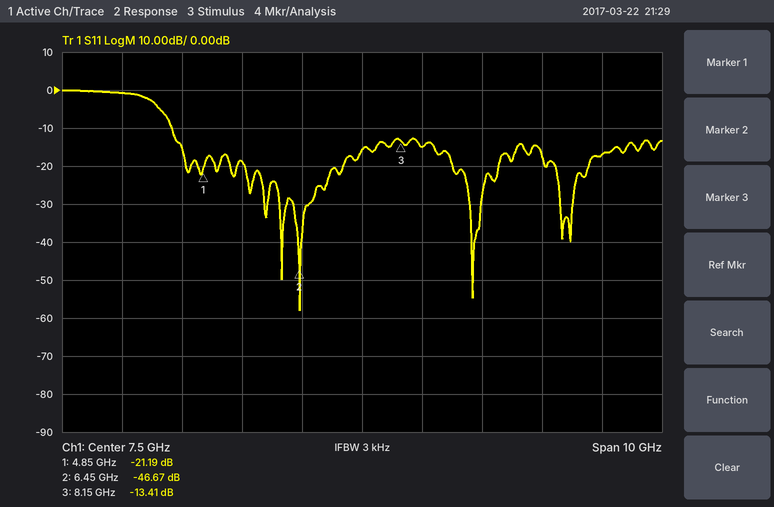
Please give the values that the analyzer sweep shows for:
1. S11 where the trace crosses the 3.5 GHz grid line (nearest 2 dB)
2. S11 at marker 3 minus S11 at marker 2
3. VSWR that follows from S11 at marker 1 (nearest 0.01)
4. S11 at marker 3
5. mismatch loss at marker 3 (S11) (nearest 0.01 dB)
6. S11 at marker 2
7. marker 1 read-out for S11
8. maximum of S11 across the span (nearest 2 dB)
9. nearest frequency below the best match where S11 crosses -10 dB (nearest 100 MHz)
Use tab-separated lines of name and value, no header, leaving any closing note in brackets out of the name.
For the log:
S11 where the trace crosses the 3.5 GHz grid line	0 dB
S11 at marker 3 minus S11 at marker 2	33.26 dB
VSWR that follows from S11 at marker 1	1.19
S11 at marker 3	-13.41 dB
mismatch loss at marker 3 (S11)	0.20 dB
S11 at marker 2	-46.67 dB
marker 1 read-out for S11	-21.19 dB
maximum of S11 across the span	0 dB
nearest frequency below the best match where S11 crosses -10 dB	4.3 GHz
